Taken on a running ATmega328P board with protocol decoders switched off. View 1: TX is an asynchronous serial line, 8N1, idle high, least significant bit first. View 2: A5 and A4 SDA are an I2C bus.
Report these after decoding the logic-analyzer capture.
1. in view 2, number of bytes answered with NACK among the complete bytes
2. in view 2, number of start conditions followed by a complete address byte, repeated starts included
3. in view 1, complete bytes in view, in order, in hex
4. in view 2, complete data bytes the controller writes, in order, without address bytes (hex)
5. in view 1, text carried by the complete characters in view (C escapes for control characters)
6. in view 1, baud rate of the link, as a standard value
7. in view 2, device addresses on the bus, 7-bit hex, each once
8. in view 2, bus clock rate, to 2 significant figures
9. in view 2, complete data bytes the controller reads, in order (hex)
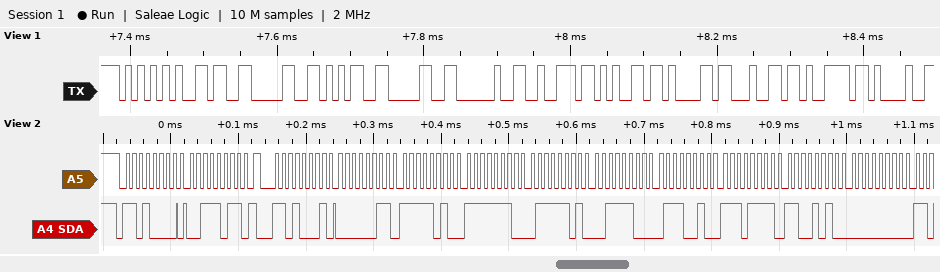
0
2
55 36 30 35 30 20 72 65 61 64 79 21
3B
"U6050 ready!"
115200 baud
0x68
100 kHz
03 FA FE 7D 3C 72 EF CA 00
